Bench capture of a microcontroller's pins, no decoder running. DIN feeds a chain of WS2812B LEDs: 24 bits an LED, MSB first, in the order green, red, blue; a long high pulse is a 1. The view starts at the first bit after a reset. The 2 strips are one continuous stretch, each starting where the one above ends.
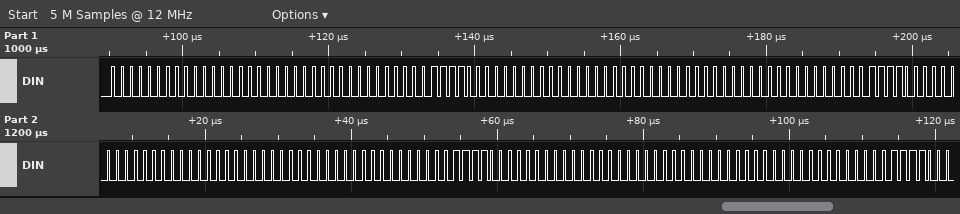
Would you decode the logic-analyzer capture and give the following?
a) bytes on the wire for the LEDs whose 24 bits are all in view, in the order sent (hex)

00 00 00 00 1E 00 00 00 00 00 1E 00 00 00 00 00 1E 00 00 00 00
